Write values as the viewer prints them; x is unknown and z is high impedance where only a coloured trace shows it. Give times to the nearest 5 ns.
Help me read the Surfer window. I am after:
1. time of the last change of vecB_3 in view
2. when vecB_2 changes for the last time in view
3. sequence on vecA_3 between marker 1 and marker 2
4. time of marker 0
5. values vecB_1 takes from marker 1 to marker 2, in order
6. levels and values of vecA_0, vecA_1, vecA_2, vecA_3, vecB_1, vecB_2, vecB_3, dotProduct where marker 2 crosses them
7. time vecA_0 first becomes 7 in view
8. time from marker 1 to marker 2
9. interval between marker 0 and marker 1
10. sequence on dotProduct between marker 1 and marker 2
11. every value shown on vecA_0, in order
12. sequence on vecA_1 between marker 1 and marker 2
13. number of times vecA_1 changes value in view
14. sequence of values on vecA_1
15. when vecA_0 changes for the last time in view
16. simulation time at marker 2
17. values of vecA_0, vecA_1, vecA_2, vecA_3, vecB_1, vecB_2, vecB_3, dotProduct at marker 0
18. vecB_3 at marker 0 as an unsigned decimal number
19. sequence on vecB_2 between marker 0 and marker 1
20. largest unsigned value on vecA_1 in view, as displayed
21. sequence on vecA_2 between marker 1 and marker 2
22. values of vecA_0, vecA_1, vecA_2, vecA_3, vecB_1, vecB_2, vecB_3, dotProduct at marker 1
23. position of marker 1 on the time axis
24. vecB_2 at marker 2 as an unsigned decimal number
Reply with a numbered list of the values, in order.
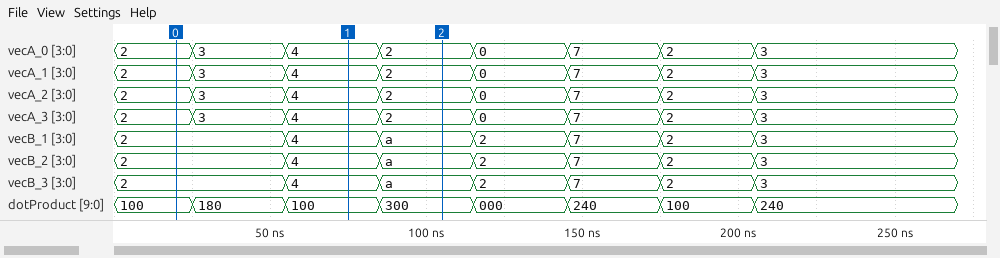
1. 205 ns
2. 205 ns
3. 4, 2
4. 20 ns
5. 4, a
6. vecA_0=2, vecA_1=2, vecA_2=2, vecA_3=2, vecB_1=a, vecB_2=a, vecB_3=a, dotProduct=300
7. 145 ns
8. 30 ns
9. 55 ns
10. 100, 300
11. 2, 3, 4, 2, 0, 7, 2, 3
12. 4, 2
13. 7
14. 2, 3, 4, 2, 0, 7, 2, 3
15. 205 ns
16. 105 ns
17. vecA_0=2, vecA_1=2, vecA_2=2, vecA_3=2, vecB_1=2, vecB_2=2, vecB_3=2, dotProduct=100
18. 2
19. 2, 4
20. 7
21. 4, 2
22. vecA_0=4, vecA_1=4, vecA_2=4, vecA_3=4, vecB_1=4, vecB_2=4, vecB_3=4, dotProduct=100
23. 75 ns
24. 10
